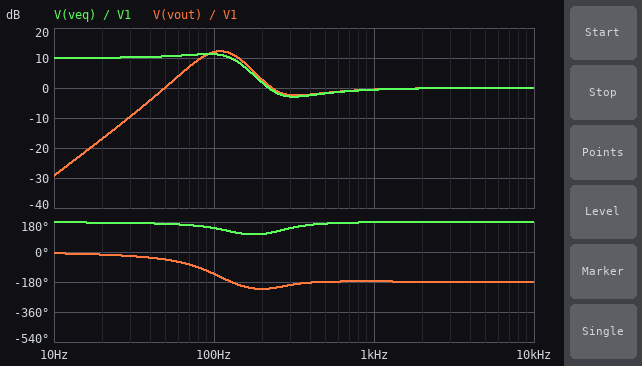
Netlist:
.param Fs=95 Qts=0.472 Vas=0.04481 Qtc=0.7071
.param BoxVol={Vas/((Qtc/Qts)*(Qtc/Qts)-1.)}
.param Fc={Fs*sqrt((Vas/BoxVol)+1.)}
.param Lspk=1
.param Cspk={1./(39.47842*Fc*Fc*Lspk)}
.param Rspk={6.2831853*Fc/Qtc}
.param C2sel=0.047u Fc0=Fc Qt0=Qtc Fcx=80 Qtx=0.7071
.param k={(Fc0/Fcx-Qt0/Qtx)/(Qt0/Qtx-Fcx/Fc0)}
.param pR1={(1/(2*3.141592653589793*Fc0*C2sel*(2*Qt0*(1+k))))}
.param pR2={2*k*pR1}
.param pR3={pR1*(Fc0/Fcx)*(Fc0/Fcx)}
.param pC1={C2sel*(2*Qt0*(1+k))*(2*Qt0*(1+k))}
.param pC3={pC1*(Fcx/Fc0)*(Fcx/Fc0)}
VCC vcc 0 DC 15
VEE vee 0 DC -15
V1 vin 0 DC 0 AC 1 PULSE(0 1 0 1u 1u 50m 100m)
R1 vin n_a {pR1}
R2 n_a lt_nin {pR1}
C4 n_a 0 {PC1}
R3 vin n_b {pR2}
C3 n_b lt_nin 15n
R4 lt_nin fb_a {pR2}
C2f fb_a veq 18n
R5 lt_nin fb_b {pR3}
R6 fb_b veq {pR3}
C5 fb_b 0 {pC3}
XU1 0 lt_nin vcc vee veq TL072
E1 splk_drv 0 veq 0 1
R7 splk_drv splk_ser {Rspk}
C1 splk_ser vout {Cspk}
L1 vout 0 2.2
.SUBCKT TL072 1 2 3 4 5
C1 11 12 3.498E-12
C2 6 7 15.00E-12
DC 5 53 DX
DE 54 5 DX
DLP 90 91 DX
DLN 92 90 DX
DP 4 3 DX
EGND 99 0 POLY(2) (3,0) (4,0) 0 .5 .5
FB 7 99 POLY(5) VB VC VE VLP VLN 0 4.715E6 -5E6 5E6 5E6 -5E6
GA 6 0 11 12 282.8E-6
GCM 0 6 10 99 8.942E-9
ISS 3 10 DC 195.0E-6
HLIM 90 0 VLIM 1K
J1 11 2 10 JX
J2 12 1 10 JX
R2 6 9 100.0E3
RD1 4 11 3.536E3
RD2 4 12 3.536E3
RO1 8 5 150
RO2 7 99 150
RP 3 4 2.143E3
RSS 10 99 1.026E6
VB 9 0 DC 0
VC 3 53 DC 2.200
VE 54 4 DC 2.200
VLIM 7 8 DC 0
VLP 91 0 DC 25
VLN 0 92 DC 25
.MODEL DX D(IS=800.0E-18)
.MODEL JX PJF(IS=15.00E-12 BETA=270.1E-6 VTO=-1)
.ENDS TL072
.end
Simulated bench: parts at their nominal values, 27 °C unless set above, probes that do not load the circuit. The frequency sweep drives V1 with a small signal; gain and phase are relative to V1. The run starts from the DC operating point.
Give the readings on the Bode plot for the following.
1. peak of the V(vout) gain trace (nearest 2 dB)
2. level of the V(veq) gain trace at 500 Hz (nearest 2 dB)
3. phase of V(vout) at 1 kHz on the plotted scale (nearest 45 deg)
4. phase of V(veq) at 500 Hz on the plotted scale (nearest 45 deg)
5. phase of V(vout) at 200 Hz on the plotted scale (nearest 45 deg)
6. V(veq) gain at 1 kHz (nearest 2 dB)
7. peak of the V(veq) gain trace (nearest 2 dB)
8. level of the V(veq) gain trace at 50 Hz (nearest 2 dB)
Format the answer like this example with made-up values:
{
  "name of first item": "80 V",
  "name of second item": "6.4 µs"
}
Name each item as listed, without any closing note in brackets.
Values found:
{
  "peak of the V(vout) gain trace": "12 dB",
  "level of the V(veq) gain trace at 500 Hz": "-2 dB",
  "phase of V(vout) at 1 kHz on the plotted scale": "-180 deg",
  "phase of V(veq) at 500 Hz on the plotted scale": "180 deg",
  "phase of V(vout) at 200 Hz on the plotted scale": "-225 deg",
  "V(veq) gain at 1 kHz": "0 dB",
  "peak of the V(veq) gain trace": "12 dB",
  "level of the V(veq) gain trace at 50 Hz": "10 dB"
}
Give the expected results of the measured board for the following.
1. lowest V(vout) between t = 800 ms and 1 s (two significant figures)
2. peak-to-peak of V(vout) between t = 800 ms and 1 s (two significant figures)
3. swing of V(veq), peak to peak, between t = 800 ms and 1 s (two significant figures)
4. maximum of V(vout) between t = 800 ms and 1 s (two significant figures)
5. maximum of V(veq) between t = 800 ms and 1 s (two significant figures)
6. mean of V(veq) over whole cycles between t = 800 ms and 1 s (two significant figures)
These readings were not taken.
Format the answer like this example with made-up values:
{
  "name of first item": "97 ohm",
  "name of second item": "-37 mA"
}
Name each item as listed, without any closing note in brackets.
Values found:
{
  "lowest V(vout) between t = 800 ms and 1 s": "-1.1 V",
  "peak-to-peak of V(vout) between t = 800 ms and 1 s": "2.3 V",
  "swing of V(veq), peak to peak, between t = 800 ms and 1 s": "4.2 V",
  "maximum of V(vout) between t = 800 ms and 1 s": "1.1 V",
  "maximum of V(veq) between t = 800 ms and 1 s": "530 mV",
  "mean of V(veq) over whole cycles between t = 800 ms and 1 s": "-1.6 V"
}
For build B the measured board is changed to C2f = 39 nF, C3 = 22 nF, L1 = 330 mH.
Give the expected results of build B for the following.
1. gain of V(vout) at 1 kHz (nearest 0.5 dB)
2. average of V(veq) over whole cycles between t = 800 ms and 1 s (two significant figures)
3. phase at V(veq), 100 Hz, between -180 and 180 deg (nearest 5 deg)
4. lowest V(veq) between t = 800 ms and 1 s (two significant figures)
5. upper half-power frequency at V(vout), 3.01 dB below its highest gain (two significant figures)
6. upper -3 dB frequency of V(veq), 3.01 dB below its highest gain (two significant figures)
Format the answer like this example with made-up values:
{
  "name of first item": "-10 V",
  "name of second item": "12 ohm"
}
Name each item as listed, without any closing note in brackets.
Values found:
{
  "gain of V(vout) at 1 kHz": "-1.5 dB",
  "average of V(veq) over whole cycles between t = 800 ms and 1 s": "-1.6 V",
  "phase at V(veq), 100 Hz, between -180 and 180 deg": "120 deg",
  "lowest V(veq) between t = 800 ms and 1 s": "-3.4 V",
  "upper half-power frequency at V(vout), 3.01 dB below its highest gain": "550 kHz",
  "upper -3 dB frequency of V(veq), 3.01 dB below its highest gain": "93 Hz"
}
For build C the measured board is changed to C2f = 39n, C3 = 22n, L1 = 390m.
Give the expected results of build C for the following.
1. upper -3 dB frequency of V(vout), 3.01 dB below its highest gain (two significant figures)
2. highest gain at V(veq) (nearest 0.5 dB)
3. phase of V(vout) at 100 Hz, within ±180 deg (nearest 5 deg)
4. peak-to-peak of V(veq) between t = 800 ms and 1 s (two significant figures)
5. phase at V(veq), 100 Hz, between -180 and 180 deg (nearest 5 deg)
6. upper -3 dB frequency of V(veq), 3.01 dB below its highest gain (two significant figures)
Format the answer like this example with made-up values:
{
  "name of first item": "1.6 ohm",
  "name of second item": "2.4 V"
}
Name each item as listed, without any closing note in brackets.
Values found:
{
  "upper -3 dB frequency of V(vout), 3.01 dB below its highest gain": "550 kHz",
  "highest gain at V(veq)": "10.0 dB",
  "phase of V(vout) at 100 Hz, within ±180 deg": "-110 deg",
  "peak-to-peak of V(veq) between t = 800 ms and 1 s": "3.6 V",
  "phase at V(veq), 100 Hz, between -180 and 180 deg": "120 deg",
  "upper -3 dB frequency of V(veq), 3.01 dB below its highest gain": "93 Hz"
}
